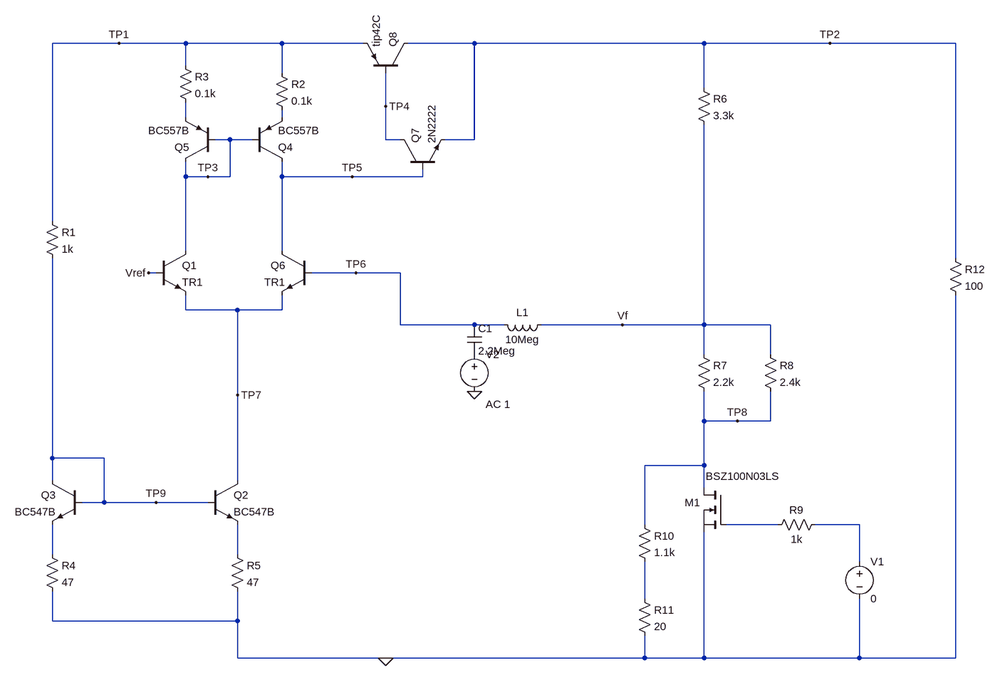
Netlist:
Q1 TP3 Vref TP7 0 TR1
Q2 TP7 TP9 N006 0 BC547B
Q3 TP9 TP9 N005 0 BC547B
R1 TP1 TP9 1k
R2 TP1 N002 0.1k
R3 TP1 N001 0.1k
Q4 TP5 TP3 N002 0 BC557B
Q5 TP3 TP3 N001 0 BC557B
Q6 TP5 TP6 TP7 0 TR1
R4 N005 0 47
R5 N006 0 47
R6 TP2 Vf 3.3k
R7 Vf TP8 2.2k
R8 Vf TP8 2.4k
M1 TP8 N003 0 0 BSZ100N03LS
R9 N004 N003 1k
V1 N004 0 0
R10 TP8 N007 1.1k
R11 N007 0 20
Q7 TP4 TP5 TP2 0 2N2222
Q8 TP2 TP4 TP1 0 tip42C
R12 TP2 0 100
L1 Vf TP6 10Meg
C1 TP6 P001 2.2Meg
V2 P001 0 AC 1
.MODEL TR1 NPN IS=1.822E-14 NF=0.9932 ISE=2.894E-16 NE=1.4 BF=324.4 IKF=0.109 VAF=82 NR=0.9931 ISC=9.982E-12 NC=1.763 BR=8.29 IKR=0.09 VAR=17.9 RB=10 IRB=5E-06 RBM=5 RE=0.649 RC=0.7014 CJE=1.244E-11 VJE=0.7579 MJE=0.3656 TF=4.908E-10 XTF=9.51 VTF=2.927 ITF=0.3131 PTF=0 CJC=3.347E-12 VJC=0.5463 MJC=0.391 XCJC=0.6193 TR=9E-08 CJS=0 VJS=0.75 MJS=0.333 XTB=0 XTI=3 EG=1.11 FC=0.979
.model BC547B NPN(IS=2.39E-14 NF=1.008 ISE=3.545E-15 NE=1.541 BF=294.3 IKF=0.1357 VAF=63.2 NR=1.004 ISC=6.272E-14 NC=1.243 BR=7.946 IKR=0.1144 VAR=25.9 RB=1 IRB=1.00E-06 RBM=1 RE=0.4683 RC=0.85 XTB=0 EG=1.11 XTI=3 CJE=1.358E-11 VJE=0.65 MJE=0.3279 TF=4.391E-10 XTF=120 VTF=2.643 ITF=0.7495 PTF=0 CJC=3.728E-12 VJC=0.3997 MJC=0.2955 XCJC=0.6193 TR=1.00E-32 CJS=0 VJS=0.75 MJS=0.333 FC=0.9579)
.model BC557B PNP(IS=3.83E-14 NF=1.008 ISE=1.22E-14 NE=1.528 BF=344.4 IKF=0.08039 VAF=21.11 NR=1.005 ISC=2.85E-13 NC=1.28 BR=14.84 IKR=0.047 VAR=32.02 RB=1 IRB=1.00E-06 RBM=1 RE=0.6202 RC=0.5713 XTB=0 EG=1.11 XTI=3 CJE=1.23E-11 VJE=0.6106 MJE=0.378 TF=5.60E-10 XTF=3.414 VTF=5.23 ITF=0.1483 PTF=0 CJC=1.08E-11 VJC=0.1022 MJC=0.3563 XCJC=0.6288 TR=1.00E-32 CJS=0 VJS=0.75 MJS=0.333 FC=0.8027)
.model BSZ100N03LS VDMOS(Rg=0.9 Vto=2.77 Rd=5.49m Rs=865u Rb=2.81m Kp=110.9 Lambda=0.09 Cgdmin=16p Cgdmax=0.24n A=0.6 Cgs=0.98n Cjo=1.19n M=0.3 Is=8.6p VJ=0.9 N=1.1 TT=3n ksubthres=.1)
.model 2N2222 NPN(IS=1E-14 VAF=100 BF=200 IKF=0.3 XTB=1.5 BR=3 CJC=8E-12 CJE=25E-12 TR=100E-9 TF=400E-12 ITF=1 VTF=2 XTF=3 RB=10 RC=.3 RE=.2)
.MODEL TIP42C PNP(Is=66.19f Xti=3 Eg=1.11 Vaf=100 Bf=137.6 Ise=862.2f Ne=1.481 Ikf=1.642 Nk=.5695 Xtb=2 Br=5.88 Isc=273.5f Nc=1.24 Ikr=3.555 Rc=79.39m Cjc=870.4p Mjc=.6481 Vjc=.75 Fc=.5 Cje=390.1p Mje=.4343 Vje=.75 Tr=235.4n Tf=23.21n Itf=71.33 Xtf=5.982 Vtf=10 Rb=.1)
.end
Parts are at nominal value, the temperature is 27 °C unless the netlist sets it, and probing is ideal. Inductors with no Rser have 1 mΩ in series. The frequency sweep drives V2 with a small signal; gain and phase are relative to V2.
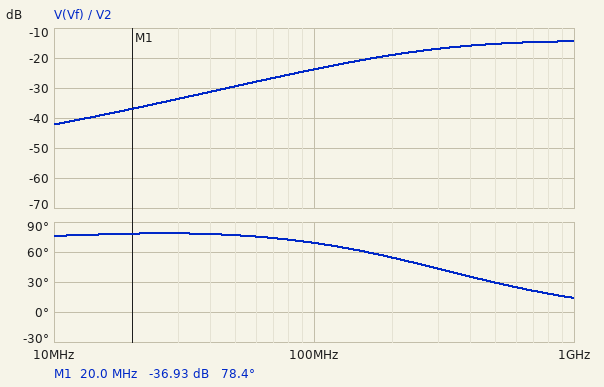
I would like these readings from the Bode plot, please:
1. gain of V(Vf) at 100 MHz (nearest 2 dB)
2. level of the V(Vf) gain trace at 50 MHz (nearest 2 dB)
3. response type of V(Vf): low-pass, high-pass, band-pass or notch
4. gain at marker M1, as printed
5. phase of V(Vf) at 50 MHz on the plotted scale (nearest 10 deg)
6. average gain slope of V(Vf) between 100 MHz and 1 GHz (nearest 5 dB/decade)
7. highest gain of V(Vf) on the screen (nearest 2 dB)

-24 dB
-30 dB
high-pass
-36.93 dB
80 deg
10 dB/decade
-14 dB
